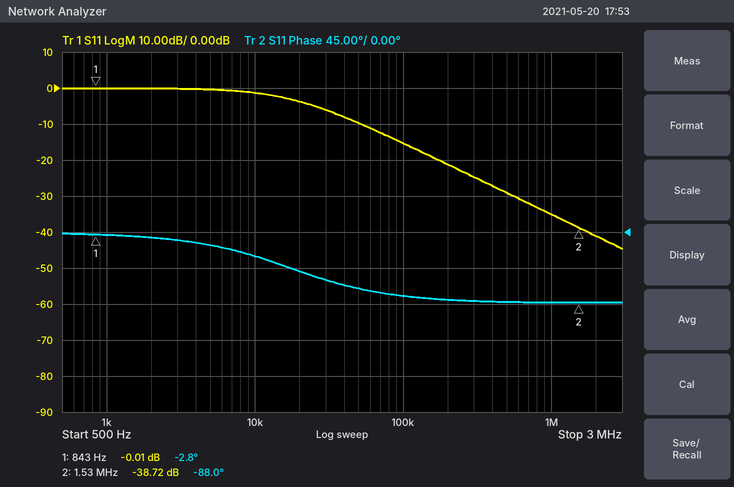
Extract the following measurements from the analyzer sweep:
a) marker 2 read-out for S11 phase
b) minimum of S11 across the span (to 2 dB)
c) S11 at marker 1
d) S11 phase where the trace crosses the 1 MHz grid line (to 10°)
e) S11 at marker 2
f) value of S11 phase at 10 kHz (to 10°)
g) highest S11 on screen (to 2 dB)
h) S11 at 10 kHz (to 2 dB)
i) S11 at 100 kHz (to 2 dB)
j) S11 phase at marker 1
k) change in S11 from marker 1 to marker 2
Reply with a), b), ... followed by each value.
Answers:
a) -88.0°
b) -44 dB
c) -0.01 dB
d) -90°
e) -38.72 dB
f) -30°
g) 0 dB
h) -2 dB
i) -16 dB
j) -2.8°
k) -38.71 dB
